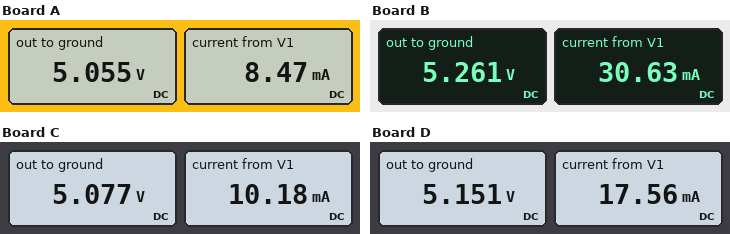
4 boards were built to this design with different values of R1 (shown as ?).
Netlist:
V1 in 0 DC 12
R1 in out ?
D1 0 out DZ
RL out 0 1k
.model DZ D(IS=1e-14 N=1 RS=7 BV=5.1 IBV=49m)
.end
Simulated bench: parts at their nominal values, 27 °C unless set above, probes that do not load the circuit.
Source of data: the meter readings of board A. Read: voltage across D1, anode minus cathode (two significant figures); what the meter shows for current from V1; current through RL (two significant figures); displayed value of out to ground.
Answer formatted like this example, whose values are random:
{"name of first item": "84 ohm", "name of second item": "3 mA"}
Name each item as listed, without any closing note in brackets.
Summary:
{"voltage across D1, anode minus cathode": "-5.1 V", "what the meter shows for current from V1": "8.47 mA", "current through RL": "5.1 mA", "displayed value of out to ground": "5.055 V"}
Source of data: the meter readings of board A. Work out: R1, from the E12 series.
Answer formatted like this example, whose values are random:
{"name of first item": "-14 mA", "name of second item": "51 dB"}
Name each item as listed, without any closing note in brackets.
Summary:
{"R1, from the E12 series": "820 Ω"}
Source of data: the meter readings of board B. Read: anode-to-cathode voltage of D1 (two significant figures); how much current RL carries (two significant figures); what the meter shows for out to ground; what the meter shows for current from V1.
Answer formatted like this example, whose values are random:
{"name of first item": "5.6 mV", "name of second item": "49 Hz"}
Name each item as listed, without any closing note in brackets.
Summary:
{"anode-to-cathode voltage of D1": "-5.3 V", "how much current RL carries": "5.3 mA", "what the meter shows for out to ground": "5.261 V", "what the meter shows for current from V1": "30.63 mA"}
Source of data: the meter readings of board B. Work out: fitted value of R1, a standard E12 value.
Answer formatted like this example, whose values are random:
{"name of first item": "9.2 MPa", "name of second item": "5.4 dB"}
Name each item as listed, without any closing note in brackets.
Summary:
{"fitted value of R1, a standard E12 value": "220 Ω"}
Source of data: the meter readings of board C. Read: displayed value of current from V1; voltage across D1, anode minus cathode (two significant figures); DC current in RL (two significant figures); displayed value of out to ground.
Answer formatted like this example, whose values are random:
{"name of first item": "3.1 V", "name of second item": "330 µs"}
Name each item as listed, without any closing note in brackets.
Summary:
{"displayed value of current from V1": "10.18 mA", "voltage across D1, anode minus cathode": "-5.1 V", "DC current in RL": "5.1 mA", "displayed value of out to ground": "5.077 V"}
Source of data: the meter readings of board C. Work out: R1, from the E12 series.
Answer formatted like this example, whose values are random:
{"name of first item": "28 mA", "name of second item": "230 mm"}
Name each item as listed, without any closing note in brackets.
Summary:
{"R1, from the E12 series": "680 Ω"}
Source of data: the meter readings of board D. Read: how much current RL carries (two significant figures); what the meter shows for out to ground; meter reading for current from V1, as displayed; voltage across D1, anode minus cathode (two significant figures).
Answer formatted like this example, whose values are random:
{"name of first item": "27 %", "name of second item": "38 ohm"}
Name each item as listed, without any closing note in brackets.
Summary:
{"how much current RL carries": "5.2 mA", "what the meter shows for out to ground": "5.151 V", "meter reading for current from V1, as displayed": "17.56 mA", "voltage across D1, anode minus cathode": "-5.2 V"}
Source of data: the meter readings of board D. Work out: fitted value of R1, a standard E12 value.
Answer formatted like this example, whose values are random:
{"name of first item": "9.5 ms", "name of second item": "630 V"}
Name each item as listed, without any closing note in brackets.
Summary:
{"fitted value of R1, a standard E12 value": "390 Ω"}
